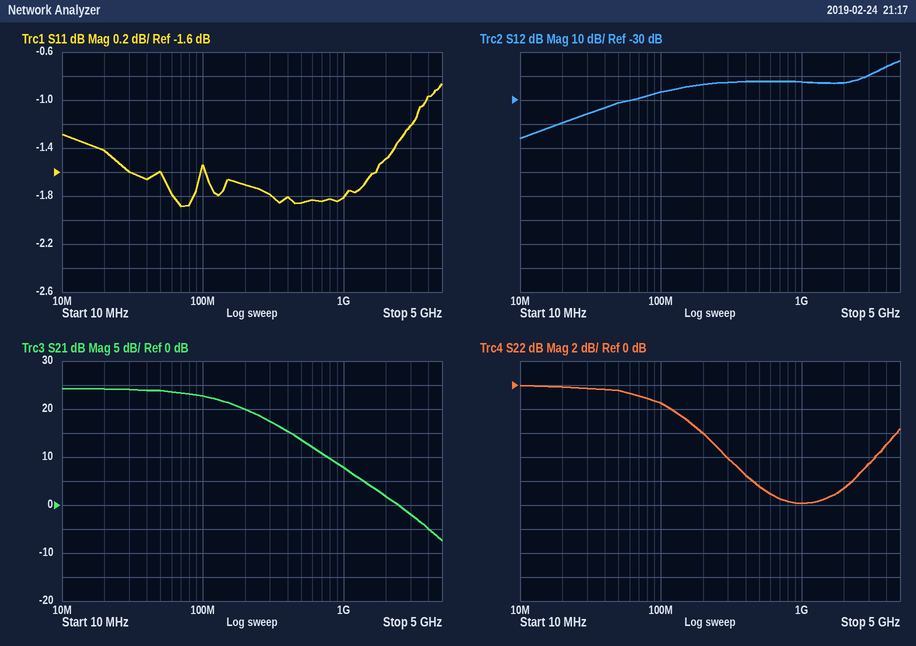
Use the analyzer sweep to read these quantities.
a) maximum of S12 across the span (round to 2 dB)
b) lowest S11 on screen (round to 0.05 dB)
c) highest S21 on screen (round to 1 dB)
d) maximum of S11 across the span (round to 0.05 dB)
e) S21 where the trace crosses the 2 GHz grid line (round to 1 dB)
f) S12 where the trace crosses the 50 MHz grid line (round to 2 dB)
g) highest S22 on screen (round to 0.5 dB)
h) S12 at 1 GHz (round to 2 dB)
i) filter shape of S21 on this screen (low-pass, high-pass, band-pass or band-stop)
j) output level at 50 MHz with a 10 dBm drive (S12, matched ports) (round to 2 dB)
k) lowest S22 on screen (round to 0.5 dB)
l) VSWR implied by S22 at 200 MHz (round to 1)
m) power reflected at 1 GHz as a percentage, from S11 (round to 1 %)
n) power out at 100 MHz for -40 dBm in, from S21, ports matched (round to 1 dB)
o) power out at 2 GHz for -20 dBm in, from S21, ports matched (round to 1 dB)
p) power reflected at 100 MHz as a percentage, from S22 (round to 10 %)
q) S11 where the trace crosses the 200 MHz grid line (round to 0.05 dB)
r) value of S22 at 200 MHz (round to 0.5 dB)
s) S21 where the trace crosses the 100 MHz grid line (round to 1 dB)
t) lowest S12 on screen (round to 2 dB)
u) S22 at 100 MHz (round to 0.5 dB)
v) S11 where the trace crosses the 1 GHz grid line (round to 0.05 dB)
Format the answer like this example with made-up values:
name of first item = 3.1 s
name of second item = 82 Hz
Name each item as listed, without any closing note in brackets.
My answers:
maximum of S12 across the span = -14 dB
lowest S11 on screen = -1.90 dB
highest S21 on screen = 24 dB
maximum of S11 across the span = -0.85 dB
S21 where the trace crosses the 2 GHz grid line = 2 dB
S12 where the trace crosses the 50 MHz grid line = -32 dB
highest S22 on screen = 0.0 dB
S12 at 1 GHz = -22 dB
filter shape of S21 on this screen = low-pass
output level at 50 MHz with a 10 dBm drive (S12, matched ports) = -22 dBm
lowest S22 on screen = -10.0 dB
VSWR implied by S22 at 200 MHz = 4
power reflected at 1 GHz as a percentage, from S11 = 66 %
power out at 100 MHz for -40 dBm in, from S21, ports matched = -17 dBm
power out at 2 GHz for -20 dBm in, from S21, ports matched = -18 dBm
power reflected at 100 MHz as a percentage, from S22 = 70 %
S11 where the trace crosses the 200 MHz grid line = -1.70 dB
value of S22 at 200 MHz = -4.0 dB
S21 where the trace crosses the 100 MHz grid line = 23 dB
lowest S12 on screen = -46 dB
S22 at 100 MHz = -1.5 dB
S11 where the trace crosses the 1 GHz grid line = -1.80 dB
